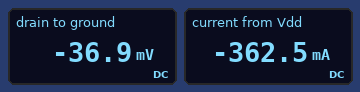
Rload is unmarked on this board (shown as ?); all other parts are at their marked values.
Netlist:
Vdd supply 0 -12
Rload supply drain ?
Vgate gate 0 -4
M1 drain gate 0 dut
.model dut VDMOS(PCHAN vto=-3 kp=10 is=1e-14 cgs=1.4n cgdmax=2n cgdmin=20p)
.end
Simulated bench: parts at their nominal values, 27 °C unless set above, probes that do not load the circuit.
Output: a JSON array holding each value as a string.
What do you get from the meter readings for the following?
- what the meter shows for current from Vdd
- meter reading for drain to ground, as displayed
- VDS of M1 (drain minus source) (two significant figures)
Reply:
["-362.5 mA", "-36.9 mV", "-37 mV"]
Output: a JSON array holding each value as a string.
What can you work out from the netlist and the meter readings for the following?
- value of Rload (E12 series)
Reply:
["33 Ω"]
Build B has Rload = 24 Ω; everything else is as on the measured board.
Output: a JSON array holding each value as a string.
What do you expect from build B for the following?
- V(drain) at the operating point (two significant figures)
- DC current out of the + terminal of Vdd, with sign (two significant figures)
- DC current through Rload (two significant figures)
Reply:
["-51 mV", "-500 mA", "500 mA"]
